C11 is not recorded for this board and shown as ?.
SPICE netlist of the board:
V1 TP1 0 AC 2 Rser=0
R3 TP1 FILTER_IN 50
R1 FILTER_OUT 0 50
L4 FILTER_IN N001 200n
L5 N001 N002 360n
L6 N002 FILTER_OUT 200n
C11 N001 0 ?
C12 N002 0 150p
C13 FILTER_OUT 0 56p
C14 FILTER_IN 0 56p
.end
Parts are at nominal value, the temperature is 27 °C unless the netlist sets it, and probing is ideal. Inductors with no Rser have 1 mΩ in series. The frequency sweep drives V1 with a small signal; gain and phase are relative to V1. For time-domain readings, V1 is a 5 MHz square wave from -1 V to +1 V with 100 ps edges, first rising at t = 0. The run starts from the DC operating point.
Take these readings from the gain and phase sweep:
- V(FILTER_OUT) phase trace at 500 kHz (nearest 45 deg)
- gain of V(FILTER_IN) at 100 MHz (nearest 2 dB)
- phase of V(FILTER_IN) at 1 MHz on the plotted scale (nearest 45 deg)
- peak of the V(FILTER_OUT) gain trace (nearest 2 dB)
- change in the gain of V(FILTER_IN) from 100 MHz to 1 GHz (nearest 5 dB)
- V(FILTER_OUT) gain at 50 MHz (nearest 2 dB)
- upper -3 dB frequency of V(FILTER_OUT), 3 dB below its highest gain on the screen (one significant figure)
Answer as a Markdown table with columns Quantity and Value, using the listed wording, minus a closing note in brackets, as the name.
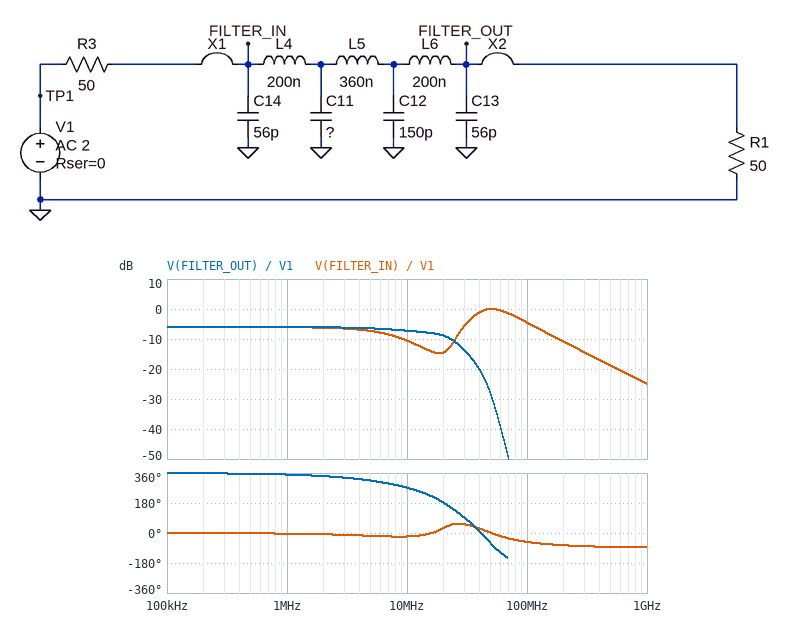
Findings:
| Quantity | Value |
|---|---|
| V(FILTER_OUT) phase trace at 500 kHz | 360 deg |
| gain of V(FILTER_IN) at 100 MHz | -4 dB |
| phase of V(FILTER_IN) at 1 MHz on the plotted scale | 0 deg |
| peak of the V(FILTER_OUT) gain trace | -6 dB |
| change in the gain of V(FILTER_IN) from 100 MHz to 1 GHz | -20 dB |
| V(FILTER_OUT) gain at 50 MHz | -28 dB |
| upper -3 dB frequency of V(FILTER_OUT), 3 dB below its highest gain on the screen | 20 MHz |
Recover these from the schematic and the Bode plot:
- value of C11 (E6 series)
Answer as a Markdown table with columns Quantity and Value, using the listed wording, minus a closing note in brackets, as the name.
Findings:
| Quantity | Value |
|---|---|
| value of C11 | 470 pF |
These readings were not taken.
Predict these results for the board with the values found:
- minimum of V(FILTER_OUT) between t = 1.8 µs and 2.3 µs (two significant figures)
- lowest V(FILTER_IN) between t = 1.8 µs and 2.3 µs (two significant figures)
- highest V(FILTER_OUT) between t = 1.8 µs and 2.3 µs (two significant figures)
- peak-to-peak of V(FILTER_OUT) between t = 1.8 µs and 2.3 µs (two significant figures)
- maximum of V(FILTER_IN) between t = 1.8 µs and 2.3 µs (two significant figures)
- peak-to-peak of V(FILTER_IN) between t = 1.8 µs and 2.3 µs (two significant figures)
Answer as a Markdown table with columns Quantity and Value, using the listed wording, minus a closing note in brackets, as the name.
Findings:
| Quantity | Value |
|---|---|
| minimum of V(FILTER_OUT) between t = 1.8 µs and 2.3 µs | -500 mV |
| lowest V(FILTER_IN) between t = 1.8 µs and 2.3 µs | -700 mV |
| highest V(FILTER_OUT) between t = 1.8 µs and 2.3 µs | 500 mV |
| peak-to-peak of V(FILTER_OUT) between t = 1.8 µs and 2.3 µs | 1.0 V |
| maximum of V(FILTER_IN) between t = 1.8 µs and 2.3 µs | 700 mV |
| peak-to-peak of V(FILTER_IN) between t = 1.8 µs and 2.3 µs | 1.4 V |
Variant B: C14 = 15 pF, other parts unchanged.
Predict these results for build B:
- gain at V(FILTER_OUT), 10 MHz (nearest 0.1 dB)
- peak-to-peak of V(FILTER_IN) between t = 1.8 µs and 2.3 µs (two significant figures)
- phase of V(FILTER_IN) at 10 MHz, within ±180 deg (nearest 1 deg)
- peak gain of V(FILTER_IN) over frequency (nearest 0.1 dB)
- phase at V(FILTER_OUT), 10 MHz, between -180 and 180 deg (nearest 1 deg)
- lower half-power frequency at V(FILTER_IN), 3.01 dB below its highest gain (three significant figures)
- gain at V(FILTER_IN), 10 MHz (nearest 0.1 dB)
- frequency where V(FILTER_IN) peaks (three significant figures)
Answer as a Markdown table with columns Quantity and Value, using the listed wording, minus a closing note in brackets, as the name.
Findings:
| Quantity | Value |
|---|---|
| gain at V(FILTER_OUT), 10 MHz | -7.1 dB |
| peak-to-peak of V(FILTER_IN) between t = 1.8 µs and 2.3 µs | 2.1 V |
| phase of V(FILTER_IN) at 10 MHz, within ±180 deg | -19 deg |
| peak gain of V(FILTER_IN) over frequency | 0 dB |
| phase at V(FILTER_OUT), 10 MHz, between -180 and 180 deg | -86 deg |
| lower half-power frequency at V(FILTER_IN), 3.01 dB below its highest gain | 41.0 MHz |
| gain at V(FILTER_IN), 10 MHz | -10.4 dB |
| frequency where V(FILTER_IN) peaks | 93.4 MHz |
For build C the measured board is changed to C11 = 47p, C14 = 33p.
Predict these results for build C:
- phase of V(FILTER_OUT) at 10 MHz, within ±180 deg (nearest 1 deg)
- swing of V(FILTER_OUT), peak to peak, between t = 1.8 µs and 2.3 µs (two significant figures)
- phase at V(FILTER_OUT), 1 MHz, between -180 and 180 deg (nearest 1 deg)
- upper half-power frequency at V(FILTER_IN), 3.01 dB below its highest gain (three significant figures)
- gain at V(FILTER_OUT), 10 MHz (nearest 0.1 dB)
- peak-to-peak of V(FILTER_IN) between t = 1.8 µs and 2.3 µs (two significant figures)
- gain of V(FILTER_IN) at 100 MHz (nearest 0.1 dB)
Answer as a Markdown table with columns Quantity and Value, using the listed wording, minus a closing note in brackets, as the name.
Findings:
| Quantity | Value |
|---|---|
| phase of V(FILTER_OUT) at 10 MHz, within ±180 deg | -54 deg |
| swing of V(FILTER_OUT), peak to peak, between t = 1.8 µs and 2.3 µs | 1.1 V |
| phase at V(FILTER_OUT), 1 MHz, between -180 and 180 deg | -5 deg |
| upper half-power frequency at V(FILTER_IN), 3.01 dB below its highest gain | 132 MHz |
| gain at V(FILTER_OUT), 10 MHz | -6.1 dB |
| peak-to-peak of V(FILTER_IN) between t = 1.8 µs and 2.3 µs | 1.7 V |
| gain of V(FILTER_IN) at 100 MHz | -0.8 dB |
